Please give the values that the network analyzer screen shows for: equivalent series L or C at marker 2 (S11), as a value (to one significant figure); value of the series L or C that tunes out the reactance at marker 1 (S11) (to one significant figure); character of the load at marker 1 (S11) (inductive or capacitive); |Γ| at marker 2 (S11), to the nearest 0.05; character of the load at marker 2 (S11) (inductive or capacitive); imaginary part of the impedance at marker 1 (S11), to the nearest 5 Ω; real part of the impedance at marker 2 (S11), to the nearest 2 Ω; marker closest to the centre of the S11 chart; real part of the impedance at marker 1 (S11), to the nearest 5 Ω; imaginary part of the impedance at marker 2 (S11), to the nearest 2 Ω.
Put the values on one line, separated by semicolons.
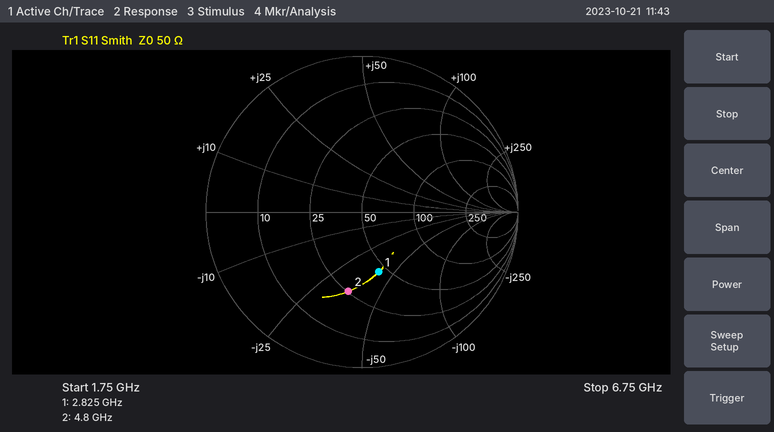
900 fF; 2 nH; capacitive; 0.50; capacitive; -40 Ω; 26 Ω; marker 1; 45 Ω; -36 Ω
